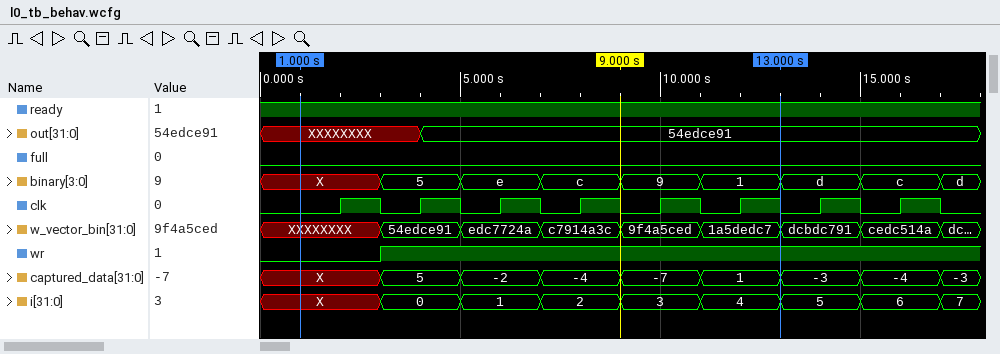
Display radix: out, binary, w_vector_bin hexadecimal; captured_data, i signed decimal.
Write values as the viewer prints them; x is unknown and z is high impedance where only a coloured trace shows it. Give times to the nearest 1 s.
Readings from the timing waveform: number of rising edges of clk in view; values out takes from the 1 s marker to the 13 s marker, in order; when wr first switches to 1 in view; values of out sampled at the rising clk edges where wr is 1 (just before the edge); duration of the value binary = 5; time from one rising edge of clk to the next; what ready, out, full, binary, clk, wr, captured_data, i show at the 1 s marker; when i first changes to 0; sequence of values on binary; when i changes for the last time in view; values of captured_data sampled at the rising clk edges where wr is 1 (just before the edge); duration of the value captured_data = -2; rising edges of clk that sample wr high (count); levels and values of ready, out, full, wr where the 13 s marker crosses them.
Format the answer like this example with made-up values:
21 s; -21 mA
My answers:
8; XXXXXXXX, 54edce91; 3 s; XXXXXXXX, 54edce91, 54edce91, 54edce91, 54edce91, 54edce91, 54edce91; 2 s; 2 s; ready=1, out=XXXXXXXX, full=0, binary=X, clk=0, wr=0, captured_data=X, i=X; 3 s; X, 5, e, c, 9, 1, d, c, d; 17 s; 5, -2, -4, -7, 1, -3, -4; 2 s; 7; ready=1, out=54edce91, full=0, wr=1
